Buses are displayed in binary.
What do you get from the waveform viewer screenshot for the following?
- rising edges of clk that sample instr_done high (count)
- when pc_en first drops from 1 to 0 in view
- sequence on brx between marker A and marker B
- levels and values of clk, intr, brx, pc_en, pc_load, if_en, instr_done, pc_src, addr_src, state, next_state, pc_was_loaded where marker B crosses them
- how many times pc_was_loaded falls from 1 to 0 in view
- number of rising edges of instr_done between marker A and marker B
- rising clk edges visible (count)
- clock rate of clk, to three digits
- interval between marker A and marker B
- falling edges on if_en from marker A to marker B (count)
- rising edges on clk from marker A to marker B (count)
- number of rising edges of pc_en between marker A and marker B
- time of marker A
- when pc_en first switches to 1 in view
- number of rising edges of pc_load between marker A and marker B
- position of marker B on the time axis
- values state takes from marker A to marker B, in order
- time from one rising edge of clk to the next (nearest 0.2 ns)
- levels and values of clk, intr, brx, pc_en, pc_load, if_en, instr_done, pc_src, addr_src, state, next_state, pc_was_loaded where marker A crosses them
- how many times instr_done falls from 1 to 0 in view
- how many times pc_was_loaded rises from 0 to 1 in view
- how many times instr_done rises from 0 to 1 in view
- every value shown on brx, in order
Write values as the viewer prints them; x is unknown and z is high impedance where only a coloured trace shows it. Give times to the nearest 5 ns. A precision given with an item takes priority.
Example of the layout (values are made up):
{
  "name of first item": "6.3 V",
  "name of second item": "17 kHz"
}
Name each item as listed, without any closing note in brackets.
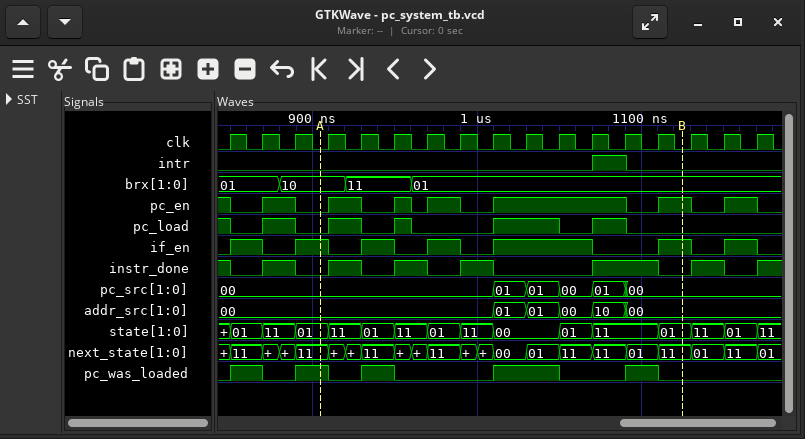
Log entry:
{
  "rising edges of clk that sample instr_done high": "8",
  "when pc_en first drops from 1 to 0 in view": "850 ns",
  "sequence on brx between marker A and marker B": "10, 11, 01",
  "levels and values of clk, intr, brx, pc_en, pc_load, if_en, instr_done, pc_src, addr_src, state, next_state, pc_was_loaded where marker B crosses them": "clk=0, intr=0, brx=01, pc_en=1, pc_load=0, if_en=1, instr_done=0, pc_src=00, addr_src=00, state=01, next_state=11, pc_was_loaded=0",
  "how many times pc_was_loaded falls from 1 to 0 in view": "5",
  "number of rising edges of instr_done between marker A and marker B": "4",
  "rising clk edges visible": "17",
  "clock rate of clk, to three digits": "50.0 MHz",
  "interval between marker A and marker B": "220 ns",
  "falling edges on if_en from marker A to marker B": "4",
  "rising edges on clk from marker A to marker B": "11",
  "number of rising edges of pc_en between marker A and marker B": "5",
  "time of marker A": "905 ns",
  "when pc_en first switches to 1 in view": "870 ns",
  "number of rising edges of pc_load between marker A and marker B": "4",
  "position of marker B on the time axis": "1125 ns",
  "values state takes from marker A to marker B, in order": "01, 11, 01, 11, 01, 11, 00, 01, 11, 01",
  "time from one rising edge of clk to the next": "20 ns",
  "levels and values of clk, intr, brx, pc_en, pc_load, if_en, instr_done, pc_src, addr_src, state, next_state, pc_was_loaded where marker A crosses them": "clk=0, intr=0, brx=10, pc_en=0, pc_load=0, if_en=1, instr_done=0, pc_src=00, addr_src=00, state=01, next_state=11, pc_was_loaded=1",
  "how many times instr_done falls from 1 to 0 in view": "7",
  "how many times pc_was_loaded rises from 0 to 1 in view": "5",
  "how many times instr_done rises from 0 to 1 in view": "7",
  "every value shown on brx, in order": "01, 10, 11, 01"
}
